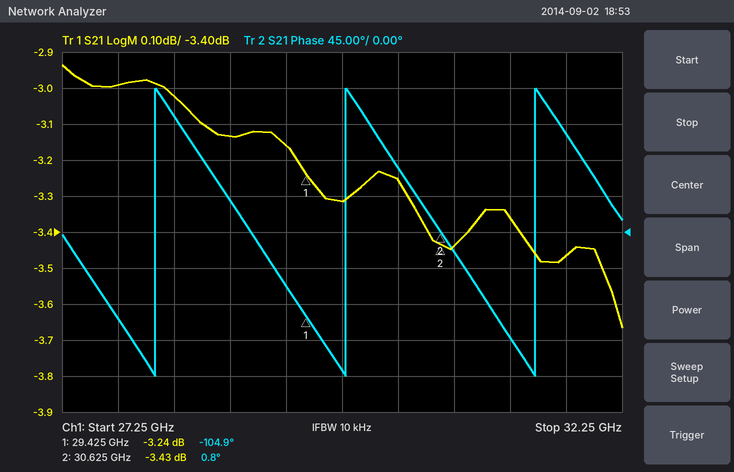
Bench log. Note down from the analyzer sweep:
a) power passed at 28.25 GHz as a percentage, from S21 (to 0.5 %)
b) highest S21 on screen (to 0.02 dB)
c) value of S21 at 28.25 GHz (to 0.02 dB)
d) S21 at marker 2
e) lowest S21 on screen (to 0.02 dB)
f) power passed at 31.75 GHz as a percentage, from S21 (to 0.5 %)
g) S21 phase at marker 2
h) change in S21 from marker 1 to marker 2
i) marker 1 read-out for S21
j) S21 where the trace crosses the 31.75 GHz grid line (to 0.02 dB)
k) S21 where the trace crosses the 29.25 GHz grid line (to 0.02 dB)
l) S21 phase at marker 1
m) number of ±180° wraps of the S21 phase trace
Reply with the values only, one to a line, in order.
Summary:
50.0 %
-2.94 dB
-3.02 dB
-3.43 dB
-3.66 dB
45.0 %
0.8°
-0.19 dB
-3.24 dB
-3.46 dB
-3.16 dB
-104.9°
3
